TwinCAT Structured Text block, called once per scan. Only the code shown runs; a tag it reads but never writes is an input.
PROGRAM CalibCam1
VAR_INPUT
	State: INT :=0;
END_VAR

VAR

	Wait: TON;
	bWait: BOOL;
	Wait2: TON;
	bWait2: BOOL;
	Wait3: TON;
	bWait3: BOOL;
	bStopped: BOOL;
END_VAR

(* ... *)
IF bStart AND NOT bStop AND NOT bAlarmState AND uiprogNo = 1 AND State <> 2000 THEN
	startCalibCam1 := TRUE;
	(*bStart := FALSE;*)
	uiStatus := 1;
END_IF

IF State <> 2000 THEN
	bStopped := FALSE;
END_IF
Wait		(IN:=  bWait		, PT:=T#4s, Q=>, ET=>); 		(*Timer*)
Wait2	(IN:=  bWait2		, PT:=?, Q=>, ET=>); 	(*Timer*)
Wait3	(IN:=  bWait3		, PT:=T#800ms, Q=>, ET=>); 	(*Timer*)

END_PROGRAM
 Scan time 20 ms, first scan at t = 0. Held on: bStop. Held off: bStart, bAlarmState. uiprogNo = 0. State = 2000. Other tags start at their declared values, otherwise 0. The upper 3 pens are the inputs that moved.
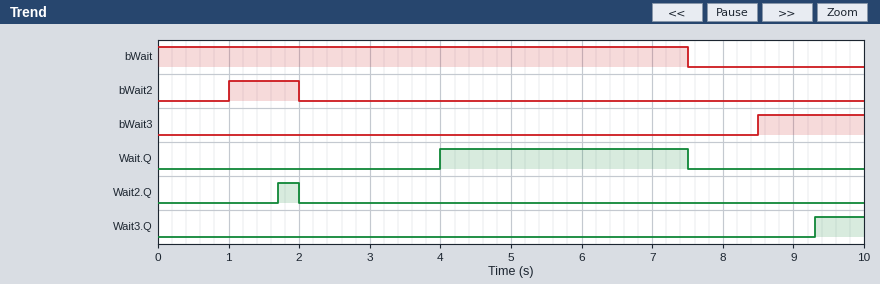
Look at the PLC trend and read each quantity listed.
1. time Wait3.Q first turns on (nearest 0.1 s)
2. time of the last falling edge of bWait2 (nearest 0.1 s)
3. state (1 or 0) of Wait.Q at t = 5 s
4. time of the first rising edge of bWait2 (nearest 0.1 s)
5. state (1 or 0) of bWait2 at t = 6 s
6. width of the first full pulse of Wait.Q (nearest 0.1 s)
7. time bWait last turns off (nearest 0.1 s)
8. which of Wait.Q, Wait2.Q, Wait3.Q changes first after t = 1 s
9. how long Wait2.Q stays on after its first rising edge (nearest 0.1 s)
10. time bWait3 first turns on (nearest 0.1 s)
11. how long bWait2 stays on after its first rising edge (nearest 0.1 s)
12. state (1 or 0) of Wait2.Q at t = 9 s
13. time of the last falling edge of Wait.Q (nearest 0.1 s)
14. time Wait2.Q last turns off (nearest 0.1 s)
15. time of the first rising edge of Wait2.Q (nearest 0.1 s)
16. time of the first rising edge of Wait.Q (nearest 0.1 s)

9.3 s
2.0 s
1
1.0 s
0
3.5 s
7.5 s
Wait2.Q
0.3 s
8.5 s
1.0 s
0
7.5 s
2.0 s
1.7 s
4.0 s
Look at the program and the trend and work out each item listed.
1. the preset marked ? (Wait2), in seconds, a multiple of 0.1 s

0.7 s
